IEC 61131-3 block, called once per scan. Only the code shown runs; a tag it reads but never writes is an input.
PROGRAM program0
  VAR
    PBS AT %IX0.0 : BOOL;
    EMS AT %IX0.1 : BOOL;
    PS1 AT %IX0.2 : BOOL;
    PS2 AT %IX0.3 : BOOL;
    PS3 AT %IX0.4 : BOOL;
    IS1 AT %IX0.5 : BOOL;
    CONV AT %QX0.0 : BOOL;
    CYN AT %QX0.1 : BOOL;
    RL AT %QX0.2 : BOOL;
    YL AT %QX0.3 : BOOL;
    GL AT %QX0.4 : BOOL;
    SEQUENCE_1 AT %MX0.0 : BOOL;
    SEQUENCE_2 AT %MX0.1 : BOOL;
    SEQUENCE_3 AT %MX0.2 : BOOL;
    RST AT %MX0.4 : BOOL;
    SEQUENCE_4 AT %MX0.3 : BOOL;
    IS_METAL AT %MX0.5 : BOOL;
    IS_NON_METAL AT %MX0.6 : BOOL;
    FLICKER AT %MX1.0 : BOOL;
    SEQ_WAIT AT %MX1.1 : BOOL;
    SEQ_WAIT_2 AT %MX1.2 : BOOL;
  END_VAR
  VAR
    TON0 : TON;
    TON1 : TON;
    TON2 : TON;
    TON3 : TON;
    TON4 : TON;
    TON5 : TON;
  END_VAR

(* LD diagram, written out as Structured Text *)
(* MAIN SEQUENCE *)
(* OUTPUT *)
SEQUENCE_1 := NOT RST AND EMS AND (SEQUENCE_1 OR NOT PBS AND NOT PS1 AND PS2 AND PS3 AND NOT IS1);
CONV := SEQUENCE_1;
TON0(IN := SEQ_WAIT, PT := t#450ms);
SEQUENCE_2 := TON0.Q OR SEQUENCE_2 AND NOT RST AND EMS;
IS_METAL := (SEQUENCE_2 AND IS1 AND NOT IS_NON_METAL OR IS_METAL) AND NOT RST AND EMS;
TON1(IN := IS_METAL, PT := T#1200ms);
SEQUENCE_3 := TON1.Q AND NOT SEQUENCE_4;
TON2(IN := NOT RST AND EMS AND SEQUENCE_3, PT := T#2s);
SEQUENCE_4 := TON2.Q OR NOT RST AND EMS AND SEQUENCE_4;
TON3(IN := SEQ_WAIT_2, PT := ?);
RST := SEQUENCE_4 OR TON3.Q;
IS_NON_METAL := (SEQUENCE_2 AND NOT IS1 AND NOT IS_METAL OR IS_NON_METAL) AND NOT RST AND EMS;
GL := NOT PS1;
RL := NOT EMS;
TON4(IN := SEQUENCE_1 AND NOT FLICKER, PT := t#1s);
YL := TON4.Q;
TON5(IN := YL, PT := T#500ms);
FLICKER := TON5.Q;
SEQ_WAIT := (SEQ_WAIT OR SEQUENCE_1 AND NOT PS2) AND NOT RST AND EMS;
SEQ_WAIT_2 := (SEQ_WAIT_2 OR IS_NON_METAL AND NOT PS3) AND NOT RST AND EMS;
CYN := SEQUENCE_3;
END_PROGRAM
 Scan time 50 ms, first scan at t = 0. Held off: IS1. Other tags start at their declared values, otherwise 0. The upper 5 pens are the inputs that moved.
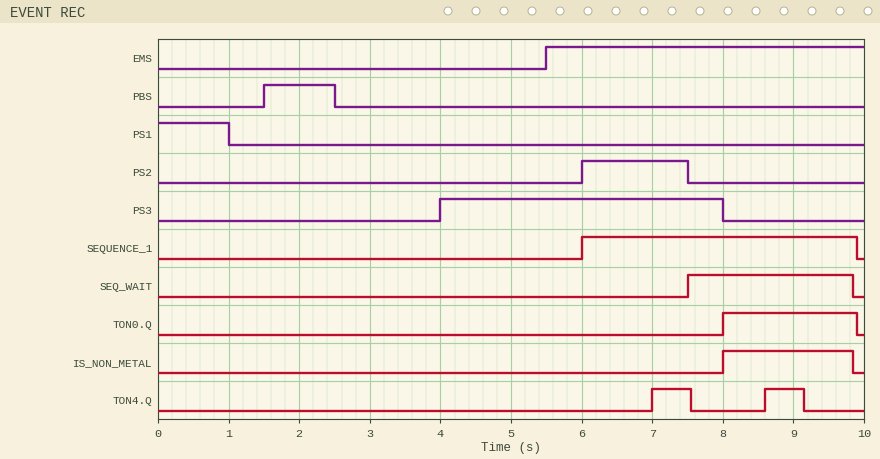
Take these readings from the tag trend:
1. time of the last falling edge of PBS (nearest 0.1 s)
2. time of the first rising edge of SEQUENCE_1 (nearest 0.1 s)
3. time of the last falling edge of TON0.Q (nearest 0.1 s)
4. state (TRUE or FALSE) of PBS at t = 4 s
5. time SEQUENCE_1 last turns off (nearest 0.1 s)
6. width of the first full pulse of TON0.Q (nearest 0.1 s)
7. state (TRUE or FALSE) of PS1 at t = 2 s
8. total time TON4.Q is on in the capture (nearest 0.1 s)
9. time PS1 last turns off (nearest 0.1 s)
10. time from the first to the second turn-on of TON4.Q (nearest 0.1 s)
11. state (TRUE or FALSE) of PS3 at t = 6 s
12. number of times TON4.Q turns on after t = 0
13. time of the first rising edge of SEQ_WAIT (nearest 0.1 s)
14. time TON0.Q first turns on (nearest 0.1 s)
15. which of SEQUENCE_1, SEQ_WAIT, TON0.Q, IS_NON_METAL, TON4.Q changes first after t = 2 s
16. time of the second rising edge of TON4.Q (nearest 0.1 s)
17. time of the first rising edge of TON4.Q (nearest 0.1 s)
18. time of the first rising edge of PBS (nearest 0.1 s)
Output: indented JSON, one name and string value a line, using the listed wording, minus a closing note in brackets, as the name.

{
  "time of the last falling edge of PBS": "2.5 s",
  "time of the first rising edge of SEQUENCE_1": "6.0 s",
  "time of the last falling edge of TON0.Q": "9.9 s",
  "state (TRUE or FALSE) of PBS at t = 4 s": "FALSE",
  "time SEQUENCE_1 last turns off": "9.9 s",
  "width of the first full pulse of TON0.Q": "1.9 s",
  "state (TRUE or FALSE) of PS1 at t = 2 s": "FALSE",
  "total time TON4.Q is on in the capture": "1.1 s",
  "time PS1 last turns off": "1.0 s",
  "time from the first to the second turn-on of TON4.Q": "1.6 s",
  "state (TRUE or FALSE) of PS3 at t = 6 s": "TRUE",
  "number of times TON4.Q turns on after t = 0": "2",
  "time of the first rising edge of SEQ_WAIT": "7.5 s",
  "time TON0.Q first turns on": "8.0 s",
  "which of SEQUENCE_1, SEQ_WAIT, TON0.Q, IS_NON_METAL, TON4.Q changes first after t = 2 s": "SEQUENCE_1",
  "time of the second rising edge of TON4.Q": "8.6 s",
  "time of the first rising edge of TON4.Q": "7.0 s",
  "time of the first rising edge of PBS": "1.5 s"
}
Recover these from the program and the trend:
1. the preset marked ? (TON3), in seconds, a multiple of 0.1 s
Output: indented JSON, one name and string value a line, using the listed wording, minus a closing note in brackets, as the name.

{
  "the preset marked ? (TON3), in seconds, a multiple of 0.1 s": "1.8 s"
}
